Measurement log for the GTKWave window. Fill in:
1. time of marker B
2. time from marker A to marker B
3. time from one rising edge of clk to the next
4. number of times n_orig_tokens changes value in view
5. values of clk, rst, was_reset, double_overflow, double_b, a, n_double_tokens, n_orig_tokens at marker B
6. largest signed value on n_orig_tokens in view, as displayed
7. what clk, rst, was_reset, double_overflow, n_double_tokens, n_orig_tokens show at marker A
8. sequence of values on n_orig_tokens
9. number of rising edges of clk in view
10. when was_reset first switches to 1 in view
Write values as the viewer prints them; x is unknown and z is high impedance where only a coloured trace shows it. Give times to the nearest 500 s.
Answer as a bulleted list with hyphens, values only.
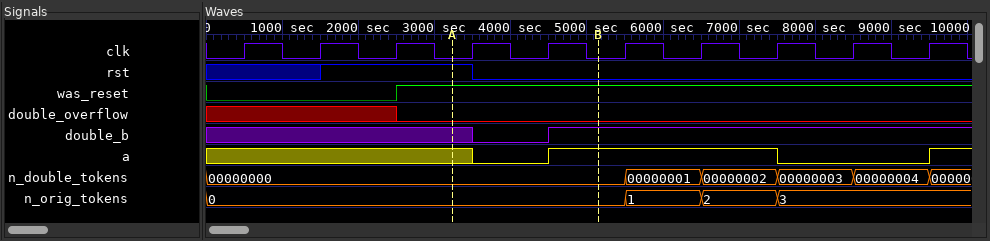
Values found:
- 5000 s
- 2000 s
- 1000 s
- 3
- clk=0, rst=0, was_reset=1, double_overflow=0, double_b=1, a=1, n_double_tokens=00000000, n_orig_tokens=0
- 3
- clk=0, rst=1, was_reset=1, double_overflow=0, n_double_tokens=00000000, n_orig_tokens=0
- 0, 1, 2, 3
- 10
- 2500 s
